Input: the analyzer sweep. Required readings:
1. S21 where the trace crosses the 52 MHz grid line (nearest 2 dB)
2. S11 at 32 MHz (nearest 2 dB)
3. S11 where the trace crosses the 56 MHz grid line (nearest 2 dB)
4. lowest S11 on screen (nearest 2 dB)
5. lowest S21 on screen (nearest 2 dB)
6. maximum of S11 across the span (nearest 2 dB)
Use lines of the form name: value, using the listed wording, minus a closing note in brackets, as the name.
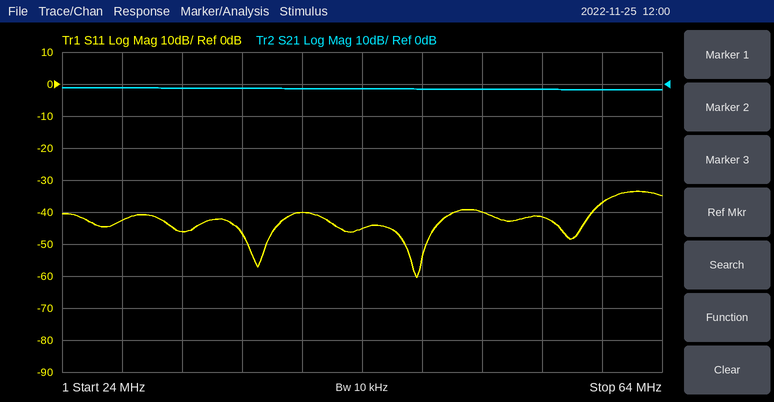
S21 where the trace crosses the 52 MHz grid line: -2 dB
S11 at 32 MHz: -46 dB
S11 where the trace crosses the 56 MHz grid line: -42 dB
lowest S11 on screen: -60 dB
lowest S21 on screen: -2 dB
maximum of S11 across the span: -34 dB
